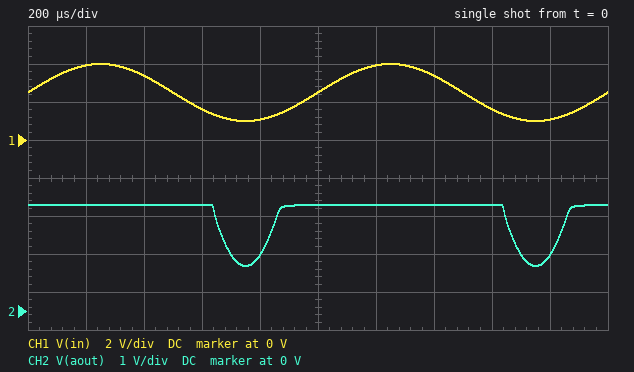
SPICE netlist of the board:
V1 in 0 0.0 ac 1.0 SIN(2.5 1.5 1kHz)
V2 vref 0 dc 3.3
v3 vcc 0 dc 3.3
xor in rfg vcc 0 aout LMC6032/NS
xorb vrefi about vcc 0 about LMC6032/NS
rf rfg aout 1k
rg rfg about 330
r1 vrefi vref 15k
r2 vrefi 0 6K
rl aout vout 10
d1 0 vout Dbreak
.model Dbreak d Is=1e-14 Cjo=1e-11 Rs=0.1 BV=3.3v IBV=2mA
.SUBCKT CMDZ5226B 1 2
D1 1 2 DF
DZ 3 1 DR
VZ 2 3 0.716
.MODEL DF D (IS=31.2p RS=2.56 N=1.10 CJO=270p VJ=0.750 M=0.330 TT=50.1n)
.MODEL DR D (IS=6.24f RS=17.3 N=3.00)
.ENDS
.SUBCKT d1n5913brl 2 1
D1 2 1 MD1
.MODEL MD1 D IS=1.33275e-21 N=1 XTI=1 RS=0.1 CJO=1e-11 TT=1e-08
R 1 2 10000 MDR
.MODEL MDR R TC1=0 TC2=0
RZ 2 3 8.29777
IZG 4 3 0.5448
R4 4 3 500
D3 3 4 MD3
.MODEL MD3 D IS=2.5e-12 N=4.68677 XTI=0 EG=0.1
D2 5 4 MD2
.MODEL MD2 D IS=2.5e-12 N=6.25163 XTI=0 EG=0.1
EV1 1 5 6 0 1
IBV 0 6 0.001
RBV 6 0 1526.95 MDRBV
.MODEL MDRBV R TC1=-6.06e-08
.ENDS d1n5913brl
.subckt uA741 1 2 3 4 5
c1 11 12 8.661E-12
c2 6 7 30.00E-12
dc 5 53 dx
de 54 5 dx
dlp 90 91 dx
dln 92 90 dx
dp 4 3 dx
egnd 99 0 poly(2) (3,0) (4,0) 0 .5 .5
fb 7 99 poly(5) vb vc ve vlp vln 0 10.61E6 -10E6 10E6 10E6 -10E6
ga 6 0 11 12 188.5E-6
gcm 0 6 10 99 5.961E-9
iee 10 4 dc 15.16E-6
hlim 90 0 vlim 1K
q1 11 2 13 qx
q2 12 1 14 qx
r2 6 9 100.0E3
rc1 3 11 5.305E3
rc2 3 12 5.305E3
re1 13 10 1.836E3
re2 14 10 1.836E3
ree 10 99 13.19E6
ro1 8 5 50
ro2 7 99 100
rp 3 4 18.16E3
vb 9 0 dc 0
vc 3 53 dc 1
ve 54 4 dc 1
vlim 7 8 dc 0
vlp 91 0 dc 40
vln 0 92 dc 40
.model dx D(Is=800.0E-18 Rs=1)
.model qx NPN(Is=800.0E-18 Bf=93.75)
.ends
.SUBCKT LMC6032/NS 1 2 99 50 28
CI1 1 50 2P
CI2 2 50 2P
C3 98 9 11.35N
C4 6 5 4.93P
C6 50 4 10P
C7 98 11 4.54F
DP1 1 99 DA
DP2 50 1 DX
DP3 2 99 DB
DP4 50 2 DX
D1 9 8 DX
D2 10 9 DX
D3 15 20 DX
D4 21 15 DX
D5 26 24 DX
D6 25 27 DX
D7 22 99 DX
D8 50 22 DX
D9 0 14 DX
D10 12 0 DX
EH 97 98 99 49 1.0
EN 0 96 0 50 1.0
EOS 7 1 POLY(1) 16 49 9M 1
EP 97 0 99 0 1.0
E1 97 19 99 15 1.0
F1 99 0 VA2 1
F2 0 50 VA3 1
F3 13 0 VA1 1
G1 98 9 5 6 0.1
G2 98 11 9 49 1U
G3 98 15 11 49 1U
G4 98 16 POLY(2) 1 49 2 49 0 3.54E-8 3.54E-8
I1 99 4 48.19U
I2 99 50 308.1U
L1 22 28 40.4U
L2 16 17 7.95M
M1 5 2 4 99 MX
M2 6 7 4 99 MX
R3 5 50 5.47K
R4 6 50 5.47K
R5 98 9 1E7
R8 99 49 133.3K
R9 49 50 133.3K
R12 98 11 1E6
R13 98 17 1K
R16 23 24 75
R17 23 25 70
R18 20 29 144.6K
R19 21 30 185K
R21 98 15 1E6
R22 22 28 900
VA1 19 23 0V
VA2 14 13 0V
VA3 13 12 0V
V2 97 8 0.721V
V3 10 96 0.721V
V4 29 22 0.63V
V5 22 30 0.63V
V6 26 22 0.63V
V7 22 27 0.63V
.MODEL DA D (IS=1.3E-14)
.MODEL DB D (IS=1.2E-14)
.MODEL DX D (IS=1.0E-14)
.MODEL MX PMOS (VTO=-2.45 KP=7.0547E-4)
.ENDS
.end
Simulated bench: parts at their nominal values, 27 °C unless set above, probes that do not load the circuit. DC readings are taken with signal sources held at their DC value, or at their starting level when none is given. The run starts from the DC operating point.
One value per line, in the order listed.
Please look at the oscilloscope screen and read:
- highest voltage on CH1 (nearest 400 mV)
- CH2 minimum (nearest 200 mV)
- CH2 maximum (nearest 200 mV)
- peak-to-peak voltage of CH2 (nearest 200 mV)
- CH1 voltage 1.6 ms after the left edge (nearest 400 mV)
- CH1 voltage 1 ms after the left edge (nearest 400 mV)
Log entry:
4.0 V
1.2 V
2.8 V
1.6 V
1.6 V
2.4 V
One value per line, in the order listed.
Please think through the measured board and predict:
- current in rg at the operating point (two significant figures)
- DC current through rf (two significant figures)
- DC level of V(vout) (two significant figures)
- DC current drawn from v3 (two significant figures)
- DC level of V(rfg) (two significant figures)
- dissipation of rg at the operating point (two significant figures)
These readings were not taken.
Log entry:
680 µA
680 µA
50 mV
1.4 mA
730 mV
150 µW
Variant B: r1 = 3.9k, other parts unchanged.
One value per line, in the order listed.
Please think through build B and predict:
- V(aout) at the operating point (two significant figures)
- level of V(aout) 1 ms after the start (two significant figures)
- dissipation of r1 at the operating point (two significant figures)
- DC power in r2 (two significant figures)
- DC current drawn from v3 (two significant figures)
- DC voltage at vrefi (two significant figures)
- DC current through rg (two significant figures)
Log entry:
91 mV
840 mV
430 µW
670 µW
1.8 mA
2.0 V
1.1 mA
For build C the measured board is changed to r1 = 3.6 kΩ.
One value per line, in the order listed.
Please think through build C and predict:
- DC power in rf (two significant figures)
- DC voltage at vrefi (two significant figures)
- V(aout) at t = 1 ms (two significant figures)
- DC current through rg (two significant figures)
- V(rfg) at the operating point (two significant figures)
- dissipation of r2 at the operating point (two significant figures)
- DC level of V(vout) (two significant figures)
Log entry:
1.2 mW
2.1 V
840 mV
1.1 mA
1.2 V
710 µW
91 mV
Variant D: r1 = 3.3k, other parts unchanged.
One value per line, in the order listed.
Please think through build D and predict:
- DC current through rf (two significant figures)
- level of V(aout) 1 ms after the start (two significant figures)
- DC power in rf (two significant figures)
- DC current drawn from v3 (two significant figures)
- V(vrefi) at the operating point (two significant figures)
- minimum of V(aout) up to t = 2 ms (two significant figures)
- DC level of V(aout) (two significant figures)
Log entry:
1.1 mA
840 mV
1.2 mW
1.8 mA
2.1 V
100 mV
91 mV
